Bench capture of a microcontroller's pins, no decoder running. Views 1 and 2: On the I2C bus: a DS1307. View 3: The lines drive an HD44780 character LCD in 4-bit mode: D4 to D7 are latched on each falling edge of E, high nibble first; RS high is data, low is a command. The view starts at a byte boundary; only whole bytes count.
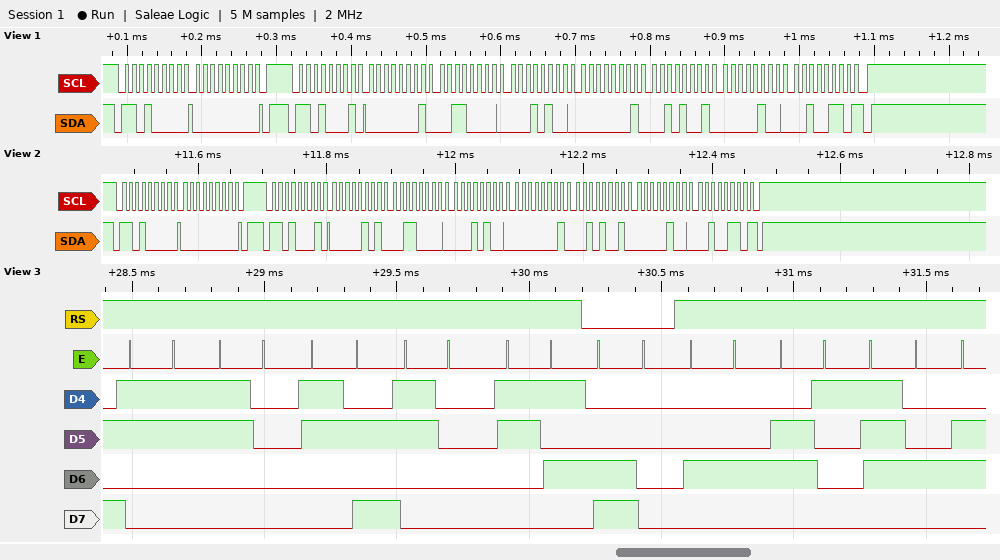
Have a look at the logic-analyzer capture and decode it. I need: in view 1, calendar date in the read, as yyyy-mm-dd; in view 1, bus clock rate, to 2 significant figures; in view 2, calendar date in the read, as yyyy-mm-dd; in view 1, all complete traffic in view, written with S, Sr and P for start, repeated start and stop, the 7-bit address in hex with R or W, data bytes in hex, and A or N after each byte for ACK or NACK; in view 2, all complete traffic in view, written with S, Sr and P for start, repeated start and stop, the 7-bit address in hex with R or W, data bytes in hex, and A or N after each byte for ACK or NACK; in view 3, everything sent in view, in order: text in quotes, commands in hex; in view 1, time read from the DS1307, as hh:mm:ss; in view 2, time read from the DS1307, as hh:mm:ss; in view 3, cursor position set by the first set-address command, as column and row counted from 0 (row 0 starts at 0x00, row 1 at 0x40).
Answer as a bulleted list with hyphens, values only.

- 2026-04-29
- 100 kHz
- 2026-04-29
- S 68W A 00 A P S 68R A 01 A 30 A 14 A 01 A 29 A 04 A 26 N P
- S 68W A 00 A P S 68R A 05 A 30 A 14 A 01 A 29 A 04 A 26 N P
- "30:05" 0xC0 "Dat"
- 14:30:01
- 14:30:05
- column 0, row 1
